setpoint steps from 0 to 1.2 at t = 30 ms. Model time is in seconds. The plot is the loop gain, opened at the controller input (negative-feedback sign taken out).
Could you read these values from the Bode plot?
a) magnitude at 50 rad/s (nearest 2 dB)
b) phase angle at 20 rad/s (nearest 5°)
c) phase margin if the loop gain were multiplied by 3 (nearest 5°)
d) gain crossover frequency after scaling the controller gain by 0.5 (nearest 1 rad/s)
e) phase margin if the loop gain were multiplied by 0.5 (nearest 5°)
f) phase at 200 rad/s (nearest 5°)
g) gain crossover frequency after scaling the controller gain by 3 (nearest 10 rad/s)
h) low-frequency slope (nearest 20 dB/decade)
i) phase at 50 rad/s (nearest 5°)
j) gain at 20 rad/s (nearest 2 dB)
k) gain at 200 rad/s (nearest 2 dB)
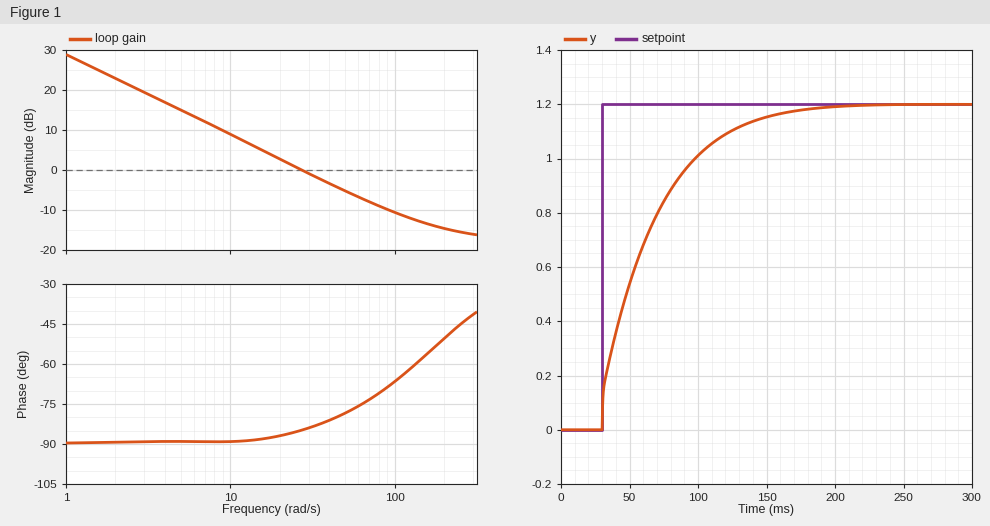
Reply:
-6 dB
-85°
110°
14 rad/s
90°
-50°
90 rad/s
-20 dB/decade
-80°
2 dB
-14 dB
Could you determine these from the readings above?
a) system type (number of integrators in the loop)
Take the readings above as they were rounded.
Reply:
1
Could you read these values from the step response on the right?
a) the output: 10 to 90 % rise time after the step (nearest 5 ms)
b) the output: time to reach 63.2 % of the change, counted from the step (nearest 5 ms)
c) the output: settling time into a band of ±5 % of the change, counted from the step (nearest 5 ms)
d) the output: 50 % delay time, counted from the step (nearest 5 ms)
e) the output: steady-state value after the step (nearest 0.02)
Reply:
85 ms
35 ms
110 ms
25 ms
1.20
